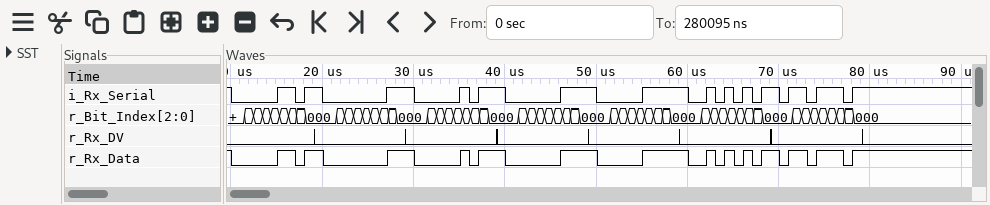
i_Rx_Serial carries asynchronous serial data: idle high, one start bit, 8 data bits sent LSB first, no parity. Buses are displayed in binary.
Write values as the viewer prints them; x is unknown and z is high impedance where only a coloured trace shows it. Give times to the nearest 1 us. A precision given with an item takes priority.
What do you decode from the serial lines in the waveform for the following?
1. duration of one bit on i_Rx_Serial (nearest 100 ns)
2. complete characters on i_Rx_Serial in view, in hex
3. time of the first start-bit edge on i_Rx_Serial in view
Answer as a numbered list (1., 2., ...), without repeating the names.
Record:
1. 1000 ns
2. B0, C0, D0, E0, F0, AA, BB
3. 10 us
